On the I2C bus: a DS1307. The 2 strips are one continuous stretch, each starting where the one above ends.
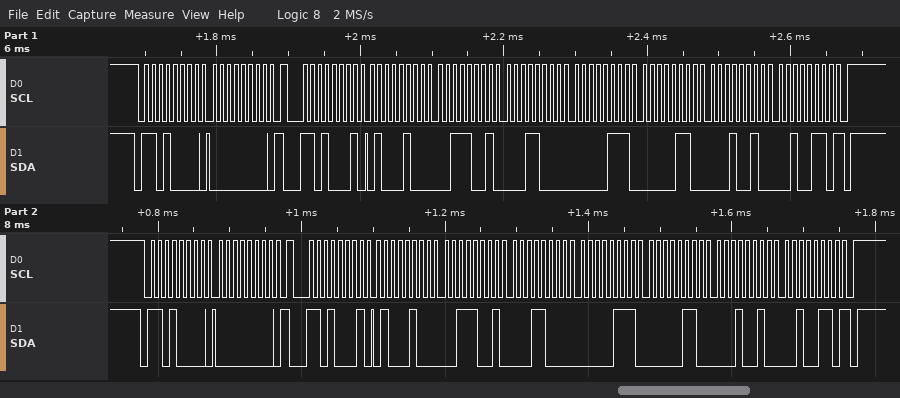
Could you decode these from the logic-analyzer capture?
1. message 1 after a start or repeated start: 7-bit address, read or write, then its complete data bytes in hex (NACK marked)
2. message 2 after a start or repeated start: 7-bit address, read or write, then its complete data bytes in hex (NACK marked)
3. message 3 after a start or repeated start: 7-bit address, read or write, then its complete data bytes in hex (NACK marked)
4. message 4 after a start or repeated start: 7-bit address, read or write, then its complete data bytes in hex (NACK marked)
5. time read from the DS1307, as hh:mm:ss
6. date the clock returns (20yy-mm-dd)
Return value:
0x68 write: 00
0x68 read: 44 39 18 07 06 12 26 NACK
0x68 write: 00
0x68 read: 44 39 18 07 06 12 26 NACK
18:39:44
2026-12-06
